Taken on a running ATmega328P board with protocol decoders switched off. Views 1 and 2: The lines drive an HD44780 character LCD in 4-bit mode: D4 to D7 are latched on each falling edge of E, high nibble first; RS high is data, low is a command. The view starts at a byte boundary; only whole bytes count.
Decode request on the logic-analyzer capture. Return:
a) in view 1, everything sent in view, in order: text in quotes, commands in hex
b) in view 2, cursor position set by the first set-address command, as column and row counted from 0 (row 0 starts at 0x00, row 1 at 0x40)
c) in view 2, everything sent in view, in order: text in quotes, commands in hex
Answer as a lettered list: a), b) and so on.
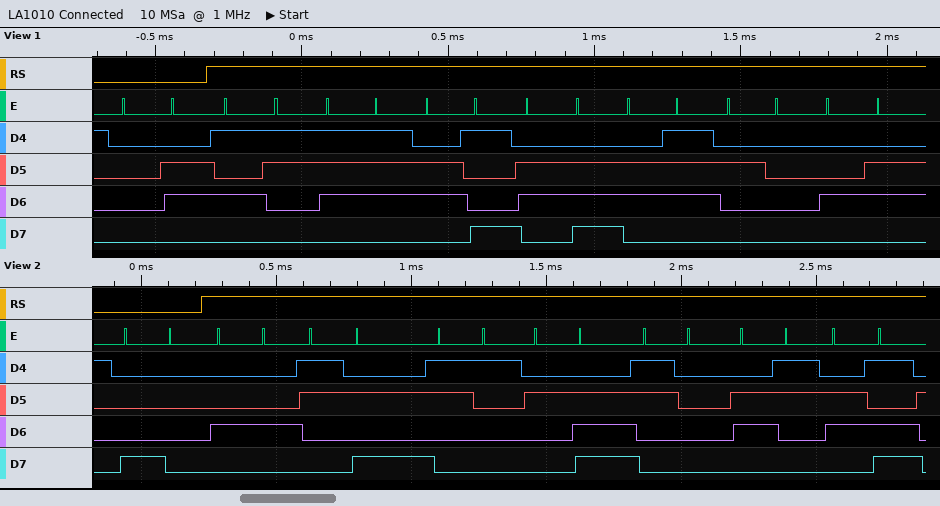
a) 0x06 "Swing F"
b) column 0, row 0
c) 0x80 "D:1.0cm"
